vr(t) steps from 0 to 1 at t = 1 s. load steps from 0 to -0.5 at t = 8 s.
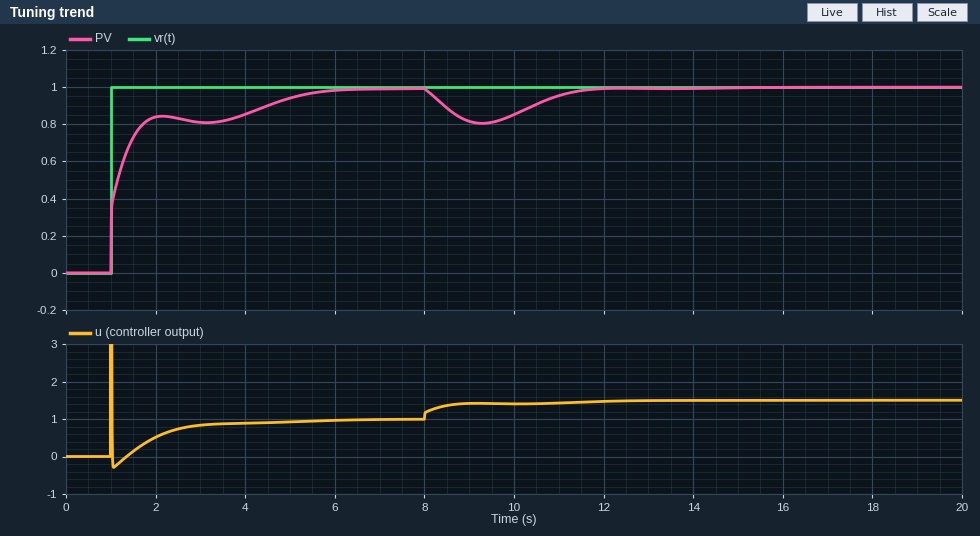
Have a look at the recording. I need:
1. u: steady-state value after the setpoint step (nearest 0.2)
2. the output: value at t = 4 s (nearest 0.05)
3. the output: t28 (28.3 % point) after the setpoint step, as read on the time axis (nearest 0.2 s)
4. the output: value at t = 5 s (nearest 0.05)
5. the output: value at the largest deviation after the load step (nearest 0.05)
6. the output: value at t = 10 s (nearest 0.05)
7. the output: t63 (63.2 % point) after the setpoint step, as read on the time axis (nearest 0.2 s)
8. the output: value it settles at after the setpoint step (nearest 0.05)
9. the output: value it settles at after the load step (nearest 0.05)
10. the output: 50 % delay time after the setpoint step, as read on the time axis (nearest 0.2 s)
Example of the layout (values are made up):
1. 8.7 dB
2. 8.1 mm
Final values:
1. 1.0
2. 0.85
3. 1.0 s
4. 0.95
5. 0.80
6. 0.85
7. 1.4 s
8. 1.00
9. 1.00
10. 1.2 s
